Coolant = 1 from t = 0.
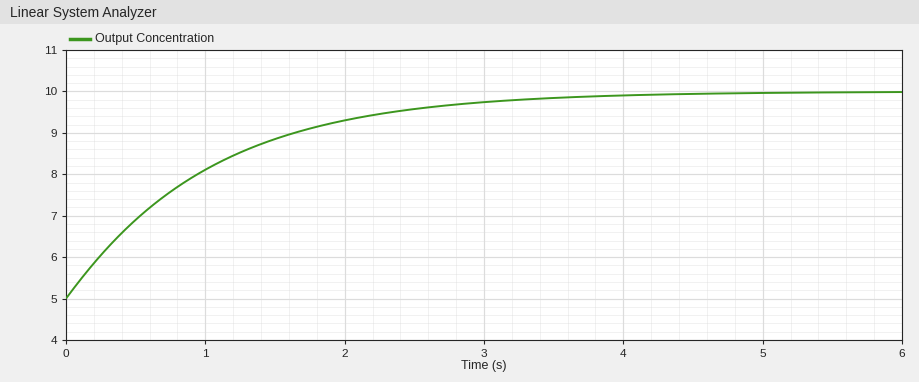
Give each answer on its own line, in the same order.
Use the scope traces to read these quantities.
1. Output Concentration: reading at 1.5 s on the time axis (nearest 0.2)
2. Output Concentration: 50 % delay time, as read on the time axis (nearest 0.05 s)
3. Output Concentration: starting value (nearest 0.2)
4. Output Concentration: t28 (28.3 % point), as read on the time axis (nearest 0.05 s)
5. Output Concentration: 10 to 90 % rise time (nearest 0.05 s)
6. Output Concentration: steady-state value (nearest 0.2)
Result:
8.8
0.70 s
5.0
0.35 s
2.20 s
10.0
